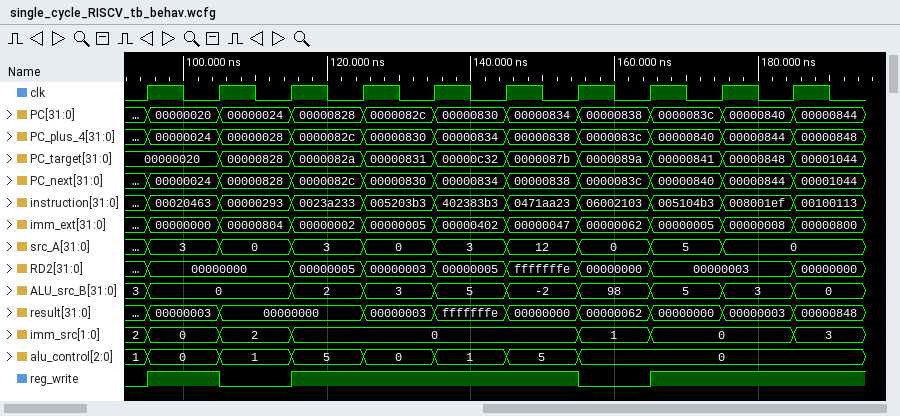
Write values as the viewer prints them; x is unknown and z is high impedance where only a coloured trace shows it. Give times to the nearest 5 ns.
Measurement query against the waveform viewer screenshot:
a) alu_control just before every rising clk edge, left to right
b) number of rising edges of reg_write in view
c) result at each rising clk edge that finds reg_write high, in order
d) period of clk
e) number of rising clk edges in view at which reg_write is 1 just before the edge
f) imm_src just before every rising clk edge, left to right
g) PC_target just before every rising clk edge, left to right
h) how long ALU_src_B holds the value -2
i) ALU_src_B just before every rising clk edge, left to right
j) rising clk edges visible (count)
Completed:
1, 0, 1, 5, 0, 1, 5, 0, 0, 0
3
00000003, 00000000, 00000003, fffffffe, 00000000, 00000000, 00000003
10 ns
7
2, 0, 2, 0, 0, 0, 0, 1, 0, 0
00000020, 00000020, 00000828, 0000082a, 00000831, 00000c32, 0000087b, 0000089a, 00000841, 00000848
10 ns
3, 0, 0, 2, 3, 5, -2, 98, 5, 3
10
